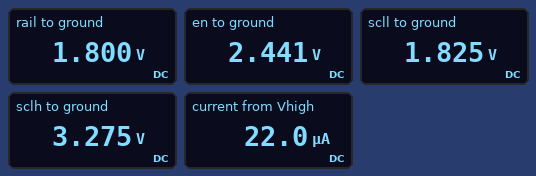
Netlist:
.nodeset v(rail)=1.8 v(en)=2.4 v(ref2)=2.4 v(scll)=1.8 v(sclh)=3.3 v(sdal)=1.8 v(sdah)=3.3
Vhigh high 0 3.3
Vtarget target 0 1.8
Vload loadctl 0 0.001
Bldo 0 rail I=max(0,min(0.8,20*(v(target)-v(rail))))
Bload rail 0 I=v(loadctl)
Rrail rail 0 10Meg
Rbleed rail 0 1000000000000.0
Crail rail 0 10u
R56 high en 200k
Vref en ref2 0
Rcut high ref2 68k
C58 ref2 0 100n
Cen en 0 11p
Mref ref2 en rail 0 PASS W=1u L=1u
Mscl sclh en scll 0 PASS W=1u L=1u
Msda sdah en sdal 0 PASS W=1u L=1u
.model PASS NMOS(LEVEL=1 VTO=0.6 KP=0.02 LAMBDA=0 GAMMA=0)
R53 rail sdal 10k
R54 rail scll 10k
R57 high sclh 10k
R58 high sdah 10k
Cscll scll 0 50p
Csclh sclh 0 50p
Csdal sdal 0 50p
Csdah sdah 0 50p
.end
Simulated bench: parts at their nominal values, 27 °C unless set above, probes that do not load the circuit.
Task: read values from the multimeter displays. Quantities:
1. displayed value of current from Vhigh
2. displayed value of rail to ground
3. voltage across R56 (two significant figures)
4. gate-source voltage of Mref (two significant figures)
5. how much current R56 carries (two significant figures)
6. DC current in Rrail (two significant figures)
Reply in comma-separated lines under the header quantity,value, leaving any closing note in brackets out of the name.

quantity,value
displayed value of current from Vhigh,22.0 µA
displayed value of rail to ground,1.800 V
voltage across R56,860 mV
gate-source voltage of Mref,640 mV
how much current R56 carries,4.3 µA
DC current in Rrail,180 nA
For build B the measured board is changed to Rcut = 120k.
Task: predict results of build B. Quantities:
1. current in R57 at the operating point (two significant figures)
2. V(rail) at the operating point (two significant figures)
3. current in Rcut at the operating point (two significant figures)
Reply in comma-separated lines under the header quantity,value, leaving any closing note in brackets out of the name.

quantity,value
current in R57 at the operating point,2.0 µA
V(rail) at the operating point,1.8 V
current in Rcut at the operating point,7.2 µA
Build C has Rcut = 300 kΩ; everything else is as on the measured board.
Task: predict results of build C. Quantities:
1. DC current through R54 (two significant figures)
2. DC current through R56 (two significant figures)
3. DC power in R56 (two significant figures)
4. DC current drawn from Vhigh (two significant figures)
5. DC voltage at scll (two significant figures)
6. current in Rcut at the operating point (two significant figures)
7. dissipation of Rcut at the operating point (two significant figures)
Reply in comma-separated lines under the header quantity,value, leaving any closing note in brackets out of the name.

quantity,value
DC current through R54,1.5 µA
DC current through R56,4.4 µA
DC power in R56,3.8 µW
DC current drawn from Vhigh,10 µA
DC voltage at scll,1.8 V
current in Rcut at the operating point,2.9 µA
dissipation of Rcut at the operating point,2.5 µW
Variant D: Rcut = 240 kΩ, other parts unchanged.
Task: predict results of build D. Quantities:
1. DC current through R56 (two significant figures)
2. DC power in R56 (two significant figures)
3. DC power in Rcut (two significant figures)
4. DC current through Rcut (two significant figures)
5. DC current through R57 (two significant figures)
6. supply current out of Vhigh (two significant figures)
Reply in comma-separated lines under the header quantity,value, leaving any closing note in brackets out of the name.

quantity,value
DC current through R56,4.4 µA
DC power in R56,3.8 µW
DC power in Rcut,3.2 µW
DC current through Rcut,3.6 µA
DC current through R57,1.6 µA
supply current out of Vhigh,11 µA
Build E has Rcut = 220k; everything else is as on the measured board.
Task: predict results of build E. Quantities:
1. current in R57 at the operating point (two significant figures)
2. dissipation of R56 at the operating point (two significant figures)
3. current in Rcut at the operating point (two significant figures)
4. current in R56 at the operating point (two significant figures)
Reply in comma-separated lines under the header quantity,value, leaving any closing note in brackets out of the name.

quantity,value
current in R57 at the operating point,1.6 µA
dissipation of R56 at the operating point,3.8 µW
current in Rcut at the operating point,4.0 µA
current in R56 at the operating point,4.4 µA
